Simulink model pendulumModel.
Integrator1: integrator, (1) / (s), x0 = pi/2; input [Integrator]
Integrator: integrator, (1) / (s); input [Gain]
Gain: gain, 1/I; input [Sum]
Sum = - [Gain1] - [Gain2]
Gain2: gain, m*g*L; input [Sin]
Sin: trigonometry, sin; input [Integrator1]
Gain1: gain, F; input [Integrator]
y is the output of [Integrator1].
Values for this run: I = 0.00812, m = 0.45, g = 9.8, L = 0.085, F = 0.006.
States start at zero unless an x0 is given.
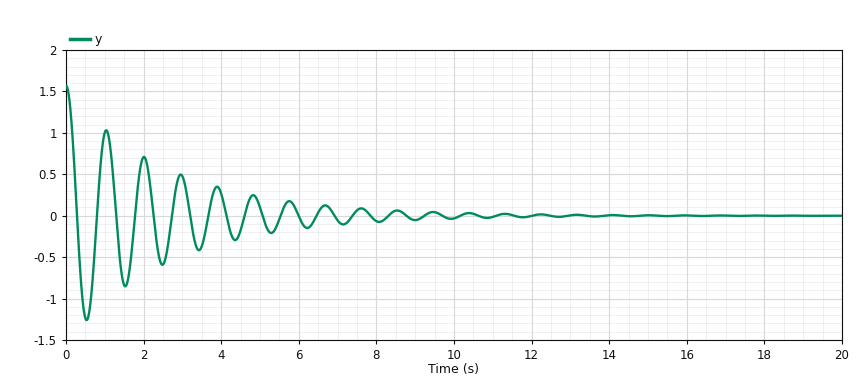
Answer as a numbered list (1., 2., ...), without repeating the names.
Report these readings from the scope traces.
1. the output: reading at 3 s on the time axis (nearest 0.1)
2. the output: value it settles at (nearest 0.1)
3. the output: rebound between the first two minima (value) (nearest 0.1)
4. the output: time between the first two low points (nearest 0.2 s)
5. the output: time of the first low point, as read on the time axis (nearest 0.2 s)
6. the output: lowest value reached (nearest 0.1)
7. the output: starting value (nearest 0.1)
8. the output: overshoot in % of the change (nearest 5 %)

1. 0.5
2. 0.0
3. 1.0
4. 1.0 s
5. 0.6 s
6. -1.3
7. 1.6
8. 80 %
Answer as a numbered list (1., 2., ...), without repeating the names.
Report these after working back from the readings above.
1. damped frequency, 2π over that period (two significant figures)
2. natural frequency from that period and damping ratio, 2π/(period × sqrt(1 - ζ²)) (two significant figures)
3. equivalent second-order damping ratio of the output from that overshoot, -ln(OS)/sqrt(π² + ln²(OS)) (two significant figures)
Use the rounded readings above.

1. 6.3 rad/s
2. 6.3 rad/s
3. 0.071
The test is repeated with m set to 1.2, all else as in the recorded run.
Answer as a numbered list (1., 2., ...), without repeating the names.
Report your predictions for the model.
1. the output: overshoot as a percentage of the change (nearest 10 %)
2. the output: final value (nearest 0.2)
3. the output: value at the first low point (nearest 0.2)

1. 90 %
2. 0.0
3. -1.4
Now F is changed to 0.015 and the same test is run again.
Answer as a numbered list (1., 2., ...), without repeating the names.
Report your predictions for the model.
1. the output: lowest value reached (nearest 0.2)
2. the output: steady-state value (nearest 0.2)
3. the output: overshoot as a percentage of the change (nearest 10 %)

1. -1.0
2. 0.0
3. 60 %
